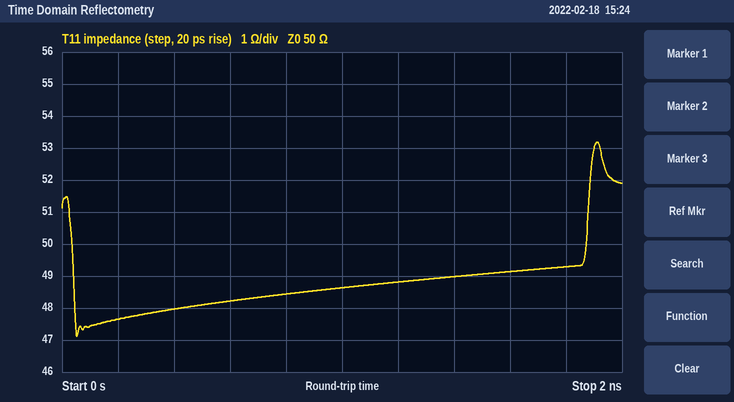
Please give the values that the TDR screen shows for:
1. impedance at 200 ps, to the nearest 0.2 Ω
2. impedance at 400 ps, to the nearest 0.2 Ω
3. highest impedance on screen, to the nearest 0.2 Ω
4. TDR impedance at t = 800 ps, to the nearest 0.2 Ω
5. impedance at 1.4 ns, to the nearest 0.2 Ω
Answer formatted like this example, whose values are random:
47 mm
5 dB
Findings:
47.6 Ω
48.0 Ω
53.2 Ω
48.4 Ω
49.0 Ω
